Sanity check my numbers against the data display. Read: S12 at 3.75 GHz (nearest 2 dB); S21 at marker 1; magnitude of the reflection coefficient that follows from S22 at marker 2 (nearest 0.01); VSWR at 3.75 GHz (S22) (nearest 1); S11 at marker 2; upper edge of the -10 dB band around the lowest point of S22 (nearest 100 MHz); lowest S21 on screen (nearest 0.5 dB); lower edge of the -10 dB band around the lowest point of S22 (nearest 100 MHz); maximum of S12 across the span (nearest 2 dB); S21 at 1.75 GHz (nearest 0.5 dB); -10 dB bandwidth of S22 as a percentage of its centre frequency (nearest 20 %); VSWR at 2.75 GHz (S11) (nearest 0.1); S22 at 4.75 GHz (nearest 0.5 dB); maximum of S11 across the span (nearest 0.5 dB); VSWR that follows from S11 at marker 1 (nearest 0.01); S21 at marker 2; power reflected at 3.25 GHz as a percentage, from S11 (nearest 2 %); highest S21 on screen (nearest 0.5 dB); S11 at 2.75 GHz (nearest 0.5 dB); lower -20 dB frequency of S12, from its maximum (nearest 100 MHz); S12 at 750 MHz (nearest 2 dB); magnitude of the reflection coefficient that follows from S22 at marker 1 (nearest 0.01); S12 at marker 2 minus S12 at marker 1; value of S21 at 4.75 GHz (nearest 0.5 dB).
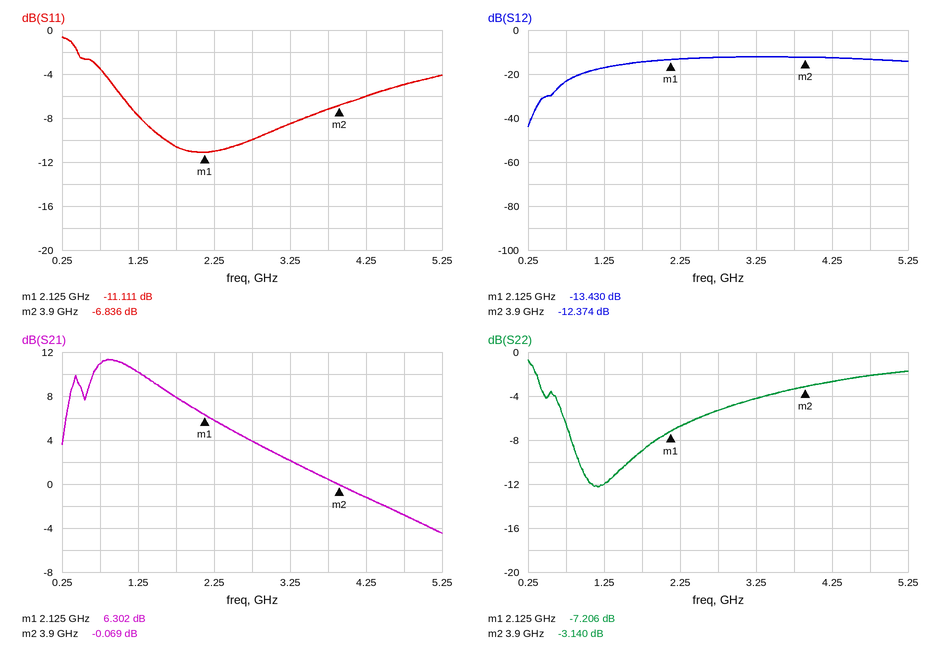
-12 dB
6.302 dB
0.70
5
-6.836 dB
1.6 GHz
-4.5 dB
900 MHz
-12 dB
8.0 dB
60 %
1.9
-2.0 dB
-0.5 dB
1.77
-0.069 dB
14 %
11.5 dB
-10.0 dB
400 MHz
-24 dB
0.44
1.056 dB
-3.0 dB
